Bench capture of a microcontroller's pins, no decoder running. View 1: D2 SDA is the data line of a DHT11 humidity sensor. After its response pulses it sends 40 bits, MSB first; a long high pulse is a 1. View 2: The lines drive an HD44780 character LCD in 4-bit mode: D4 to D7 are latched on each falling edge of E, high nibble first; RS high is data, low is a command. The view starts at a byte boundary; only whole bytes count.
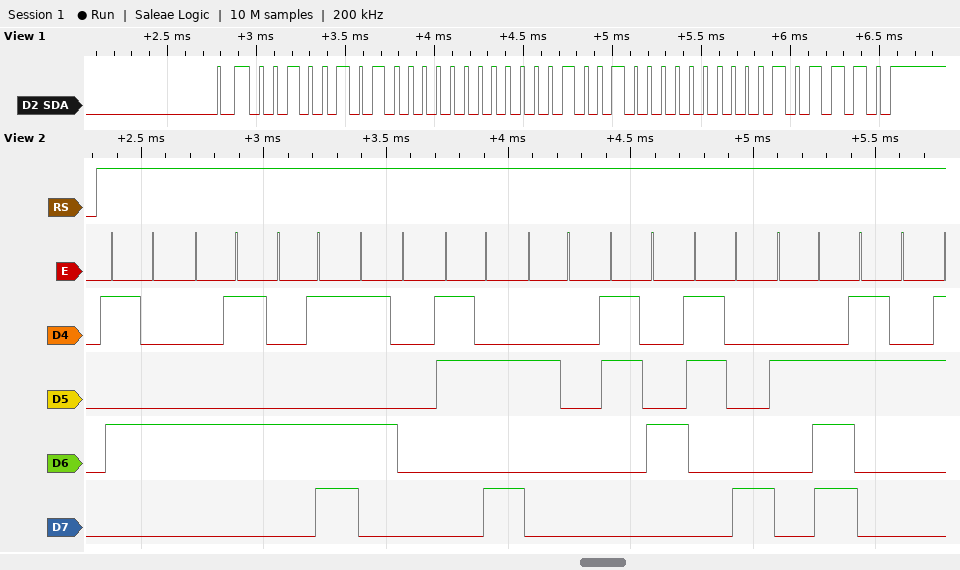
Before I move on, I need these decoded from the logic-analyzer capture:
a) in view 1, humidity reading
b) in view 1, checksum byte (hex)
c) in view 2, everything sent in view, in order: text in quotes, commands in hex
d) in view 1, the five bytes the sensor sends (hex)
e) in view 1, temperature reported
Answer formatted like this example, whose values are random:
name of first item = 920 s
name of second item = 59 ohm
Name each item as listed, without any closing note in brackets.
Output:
in view 1, humidity reading = 37 %
in view 1, checksum byte = 0x2E
in view 2, everything sent in view, in order: text in quotes, commands in hex = "TEMP: 48.2"
in view 1, the five bytes the sensor sends = 25 00 09 00 2E
in view 1, temperature reported = 9.0 °C
